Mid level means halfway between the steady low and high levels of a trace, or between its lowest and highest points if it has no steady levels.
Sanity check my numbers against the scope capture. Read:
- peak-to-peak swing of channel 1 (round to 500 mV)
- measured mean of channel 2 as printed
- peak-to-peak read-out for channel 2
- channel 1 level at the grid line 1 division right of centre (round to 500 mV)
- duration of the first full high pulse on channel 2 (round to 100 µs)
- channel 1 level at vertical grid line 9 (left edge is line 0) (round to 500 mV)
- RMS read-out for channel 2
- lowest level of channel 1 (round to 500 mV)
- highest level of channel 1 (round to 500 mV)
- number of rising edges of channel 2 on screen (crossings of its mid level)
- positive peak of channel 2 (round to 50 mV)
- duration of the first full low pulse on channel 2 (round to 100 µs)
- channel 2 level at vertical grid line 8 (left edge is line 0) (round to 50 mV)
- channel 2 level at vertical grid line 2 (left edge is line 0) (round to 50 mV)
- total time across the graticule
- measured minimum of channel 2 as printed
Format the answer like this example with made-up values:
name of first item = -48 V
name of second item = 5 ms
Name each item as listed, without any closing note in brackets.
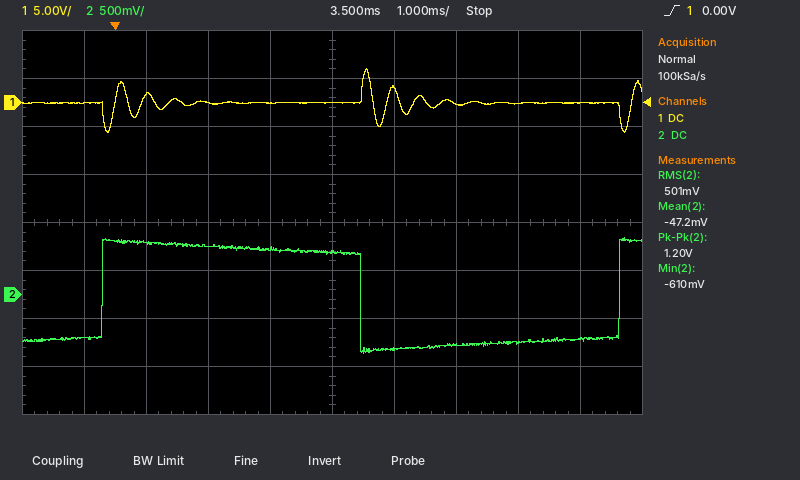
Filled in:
peak-to-peak swing of channel 1 = 6.5 V
measured mean of channel 2 as printed = -47.2 mV
peak-to-peak read-out for channel 2 = 1.20 V
channel 1 level at the grid line 1 division right of centre = 1.5 V
duration of the first full high pulse on channel 2 = 4.2 ms
channel 1 level at vertical grid line 9 (left edge is line 0) = 0.0 V
RMS read-out for channel 2 = 501 mV
lowest level of channel 1 = -3.0 V
highest level of channel 1 = 3.5 V
number of rising edges of channel 2 on screen = 2
positive peak of channel 2 = 600 mV
duration of the first full low pulse on channel 2 = 4.2 ms
channel 2 level at vertical grid line 8 (left edge is line 0) = -500 mV
channel 2 level at vertical grid line 2 (left edge is line 0) = 550 mV
total time across the graticule = 10 ms
measured minimum of channel 2 as printed = -610 mV
